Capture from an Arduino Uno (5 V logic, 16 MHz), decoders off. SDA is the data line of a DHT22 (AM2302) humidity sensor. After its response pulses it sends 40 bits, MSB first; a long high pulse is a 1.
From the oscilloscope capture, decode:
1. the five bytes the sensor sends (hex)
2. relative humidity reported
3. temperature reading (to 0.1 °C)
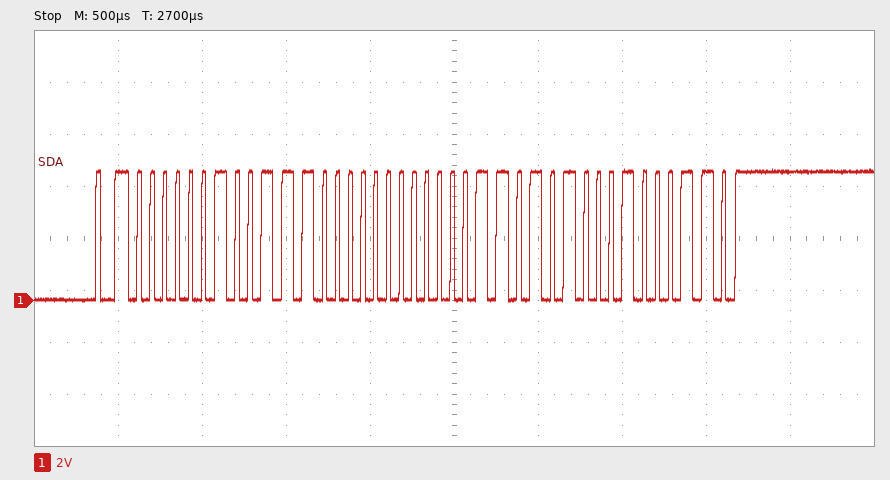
02 70 00 D4 46
62.4 %
21.2 °C
